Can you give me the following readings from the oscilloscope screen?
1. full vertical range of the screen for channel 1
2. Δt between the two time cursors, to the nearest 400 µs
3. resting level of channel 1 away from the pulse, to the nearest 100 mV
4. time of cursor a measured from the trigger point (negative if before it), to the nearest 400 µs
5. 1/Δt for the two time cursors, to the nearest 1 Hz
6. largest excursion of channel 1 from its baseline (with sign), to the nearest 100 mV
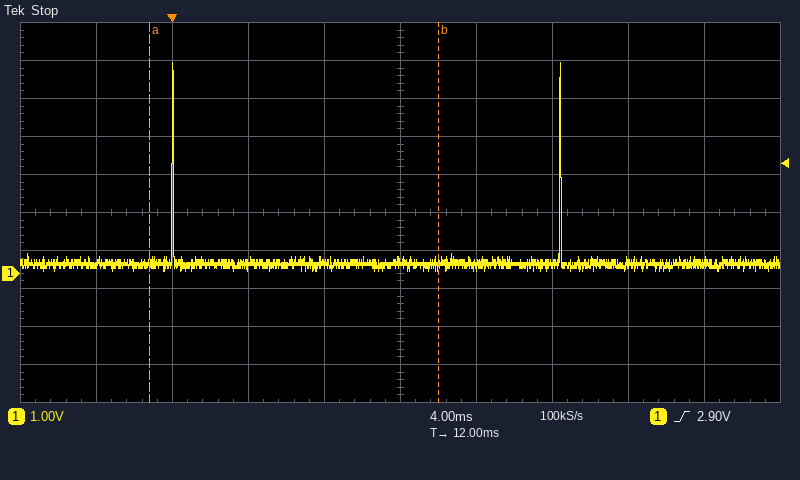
10 V
15.2 ms
200 mV
-1.2 ms
66 Hz
+5.3 V
